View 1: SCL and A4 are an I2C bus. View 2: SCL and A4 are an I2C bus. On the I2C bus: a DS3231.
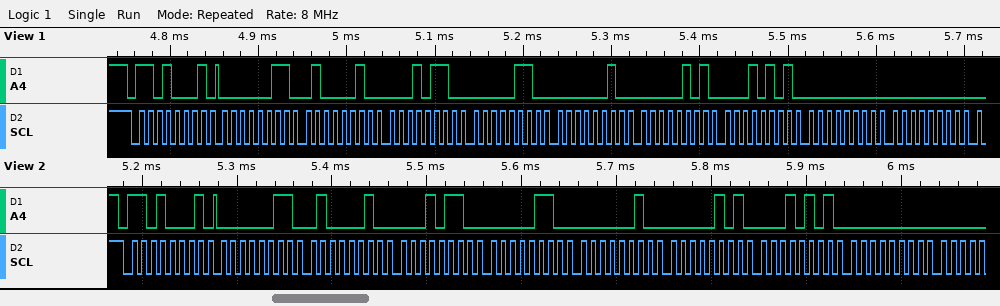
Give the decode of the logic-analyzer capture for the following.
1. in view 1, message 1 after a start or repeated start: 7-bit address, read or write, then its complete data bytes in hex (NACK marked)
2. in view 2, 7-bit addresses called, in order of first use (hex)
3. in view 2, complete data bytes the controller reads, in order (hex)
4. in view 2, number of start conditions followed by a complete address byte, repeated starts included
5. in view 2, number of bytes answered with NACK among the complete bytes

0x68 read: 03 42 16 06 02 05 15 00 00
0x68
03 42 16 06 02 05 15 00
1
0
